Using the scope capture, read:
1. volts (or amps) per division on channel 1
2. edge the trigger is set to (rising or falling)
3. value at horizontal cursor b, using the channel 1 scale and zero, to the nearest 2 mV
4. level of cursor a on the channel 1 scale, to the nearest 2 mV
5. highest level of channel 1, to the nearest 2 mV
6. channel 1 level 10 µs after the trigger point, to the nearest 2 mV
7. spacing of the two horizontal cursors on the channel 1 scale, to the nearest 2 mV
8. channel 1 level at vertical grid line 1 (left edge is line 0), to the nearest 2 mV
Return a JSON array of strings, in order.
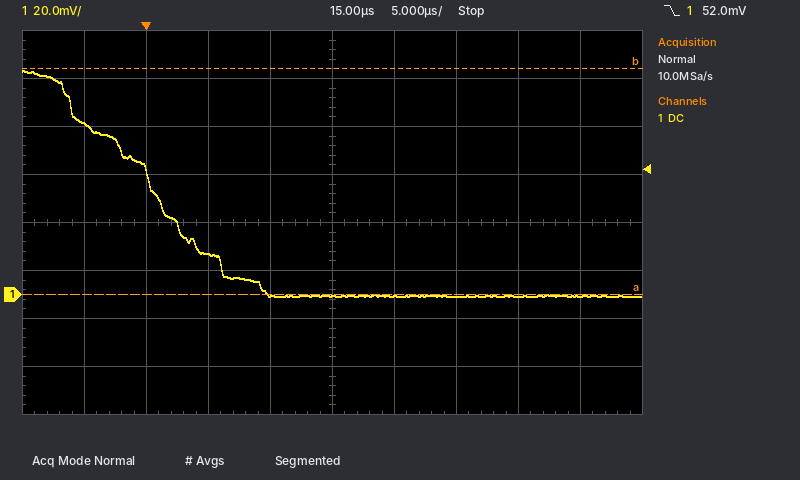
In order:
["20 mV", "falling", "94 mV", "0 mV", "94 mV", "0 mV", "94 mV", "72 mV"]
